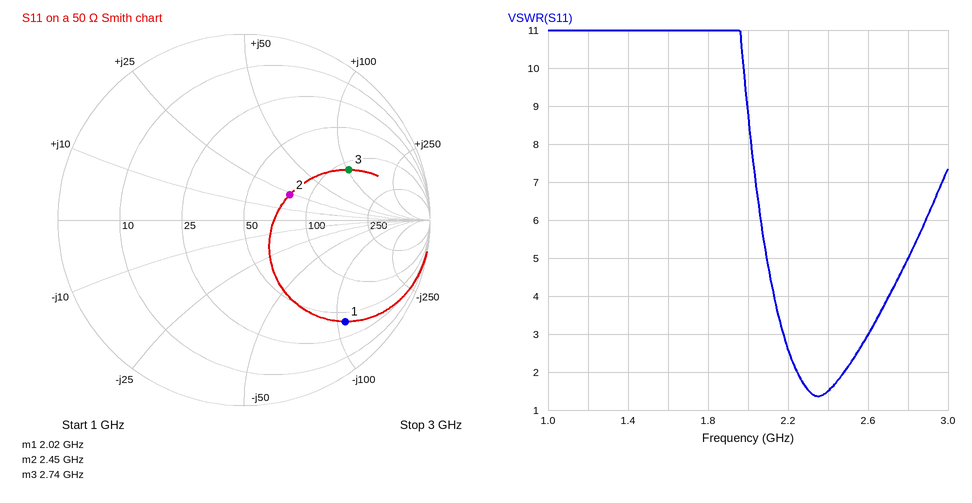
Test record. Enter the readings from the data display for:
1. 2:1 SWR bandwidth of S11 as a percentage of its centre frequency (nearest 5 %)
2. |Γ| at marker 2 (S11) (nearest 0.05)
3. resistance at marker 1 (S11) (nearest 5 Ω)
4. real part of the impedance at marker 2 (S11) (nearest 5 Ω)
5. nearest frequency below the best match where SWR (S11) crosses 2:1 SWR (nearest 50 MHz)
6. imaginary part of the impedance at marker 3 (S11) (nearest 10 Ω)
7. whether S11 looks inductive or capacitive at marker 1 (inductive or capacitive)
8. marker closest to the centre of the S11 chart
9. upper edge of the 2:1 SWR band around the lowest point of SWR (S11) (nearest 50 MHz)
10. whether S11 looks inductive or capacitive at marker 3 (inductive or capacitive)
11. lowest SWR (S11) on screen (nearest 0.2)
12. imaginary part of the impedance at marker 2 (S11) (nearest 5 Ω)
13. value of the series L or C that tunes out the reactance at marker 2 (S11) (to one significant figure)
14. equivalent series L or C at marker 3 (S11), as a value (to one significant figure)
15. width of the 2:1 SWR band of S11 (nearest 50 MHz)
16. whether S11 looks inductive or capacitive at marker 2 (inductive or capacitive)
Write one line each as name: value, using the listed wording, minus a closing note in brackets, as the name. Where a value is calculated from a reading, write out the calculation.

2:1 SWR bandwidth of S11 as a percentage of its centre frequency: 250 MHz / 2.375 GHz ≈ 10 %
|Γ| at marker 2 (S11): 0.30
resistance at marker 1 (S11): 40 Ω
real part of the impedance at marker 2 (S11): 80 Ω
nearest frequency below the best match where SWR (S11) crosses 2:1 SWR: 2.25 GHz
imaginary part of the impedance at marker 3 (S11): +100 Ω
whether S11 looks inductive or capacitive at marker 1: capacitive
marker closest to the centre of the S11 chart: marker 2
upper edge of the 2:1 SWR band around the lowest point of SWR (S11): 2.50 GHz
whether S11 looks inductive or capacitive at marker 3: inductive
lowest SWR (S11) on screen: 1.4
imaginary part of the impedance at marker 2 (S11): +25 Ω
value of the series L or C that tunes out the reactance at marker 2 (S11): C = 1/(2π × 2.45 GHz × 25 Ω) ≈ 3 pF
equivalent series L or C at marker 3 (S11), as a value: L = 100 Ω/(2π × 2.74 GHz) ≈ 6 nH
width of the 2:1 SWR band of S11: 2.50 GHz − 2.25 GHz = 250 MHz
whether S11 looks inductive or capacitive at marker 2: inductive
